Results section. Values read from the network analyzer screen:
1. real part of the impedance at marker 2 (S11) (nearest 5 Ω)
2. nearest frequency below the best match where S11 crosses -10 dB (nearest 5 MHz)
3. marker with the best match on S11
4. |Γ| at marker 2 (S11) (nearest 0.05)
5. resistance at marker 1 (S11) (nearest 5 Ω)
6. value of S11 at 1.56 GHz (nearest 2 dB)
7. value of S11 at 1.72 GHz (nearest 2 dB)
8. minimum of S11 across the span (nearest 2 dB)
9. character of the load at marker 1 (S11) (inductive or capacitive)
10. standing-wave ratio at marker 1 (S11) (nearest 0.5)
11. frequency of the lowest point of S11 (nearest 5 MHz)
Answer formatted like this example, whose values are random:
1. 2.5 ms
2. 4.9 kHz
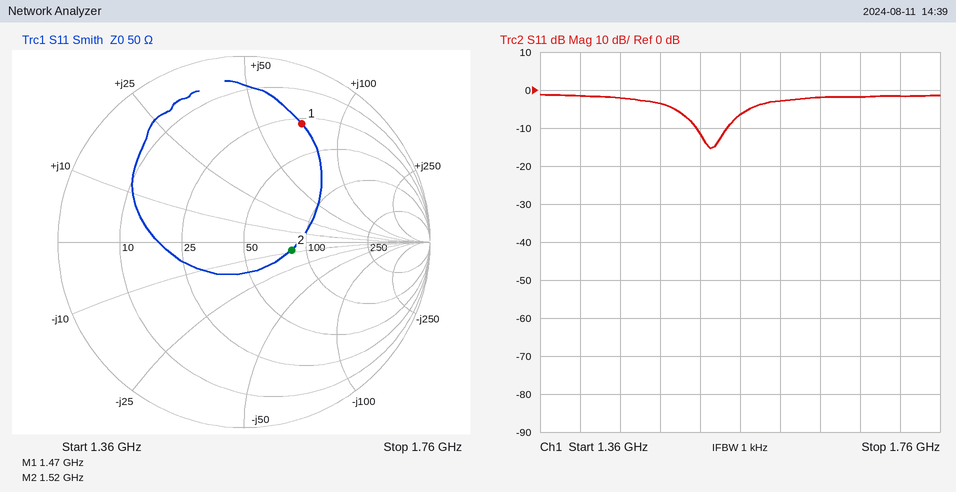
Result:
1. 85 Ω
2. 1.515 GHz
3. marker 2
4. 0.25
5. 30 Ω
6. -6 dB
7. -2 dB
8. -16 dB
9. inductive
10. 6.0
11. 1.530 GHz
